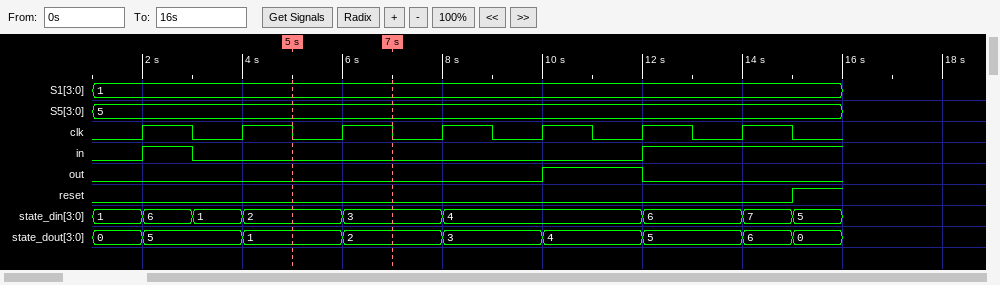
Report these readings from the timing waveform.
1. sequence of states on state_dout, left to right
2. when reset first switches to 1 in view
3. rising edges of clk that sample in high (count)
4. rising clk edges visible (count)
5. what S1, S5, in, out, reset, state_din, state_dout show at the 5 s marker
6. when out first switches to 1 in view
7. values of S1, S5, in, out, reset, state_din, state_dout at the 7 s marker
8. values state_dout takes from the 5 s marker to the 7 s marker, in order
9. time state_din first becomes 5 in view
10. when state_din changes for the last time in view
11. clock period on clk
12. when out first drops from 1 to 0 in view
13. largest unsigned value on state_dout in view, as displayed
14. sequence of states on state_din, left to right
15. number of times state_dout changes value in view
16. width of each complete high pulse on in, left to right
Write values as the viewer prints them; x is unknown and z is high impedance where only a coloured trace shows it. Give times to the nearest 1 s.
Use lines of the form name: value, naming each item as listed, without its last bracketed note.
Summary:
sequence of states on state_dout, left to right: 0, 5, 1, 2, 3, 4, 5, 6, 0
when reset first switches to 1 in view: 15 s
rising edges of clk that sample in high: 1
rising clk edges visible: 7
what S1, S5, in, out, reset, state_din, state_dout show at the 5 s marker: S1=1, S5=5, in=0, out=0, reset=0, state_din=2, state_dout=1
when out first switches to 1 in view: 10 s
values of S1, S5, in, out, reset, state_din, state_dout at the 7 s marker: S1=1, S5=5, in=0, out=0, reset=0, state_din=3, state_dout=2
values state_dout takes from the 5 s marker to the 7 s marker, in order: 1, 2
time state_din first becomes 5 in view: 15 s
when state_din changes for the last time in view: 15 s
clock period on clk: 2 s
when out first drops from 1 to 0 in view: 12 s
largest unsigned value on state_dout in view, as displayed: 6
sequence of states on state_din, left to right: 1, 6, 1, 2, 3, 4, 6, 7, 5
number of times state_dout changes value in view: 8
width of each complete high pulse on in, left to right: 1 s
